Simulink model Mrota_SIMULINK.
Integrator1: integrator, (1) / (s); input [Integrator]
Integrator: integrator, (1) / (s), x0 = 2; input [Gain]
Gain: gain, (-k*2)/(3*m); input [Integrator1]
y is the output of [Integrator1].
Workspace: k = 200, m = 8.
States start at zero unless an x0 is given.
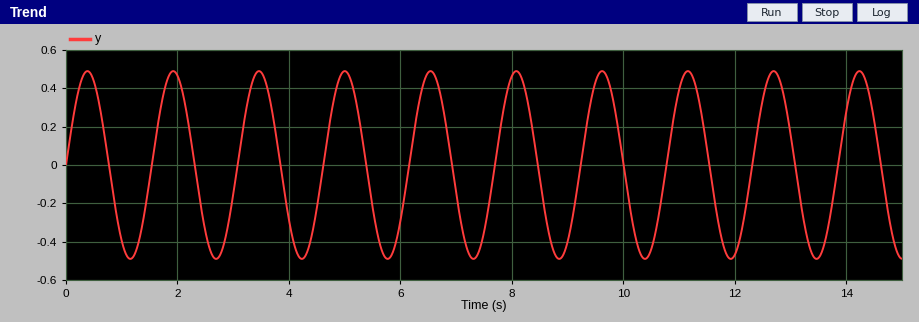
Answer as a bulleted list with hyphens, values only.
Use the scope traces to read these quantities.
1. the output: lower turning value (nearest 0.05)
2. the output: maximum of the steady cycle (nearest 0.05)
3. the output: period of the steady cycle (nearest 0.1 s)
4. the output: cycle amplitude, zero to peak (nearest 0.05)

- -0.50
- 0.50
- 1.5 s
- 0.50
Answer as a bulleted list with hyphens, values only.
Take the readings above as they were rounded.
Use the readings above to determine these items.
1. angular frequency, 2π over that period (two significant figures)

- 4.2 rad/s
